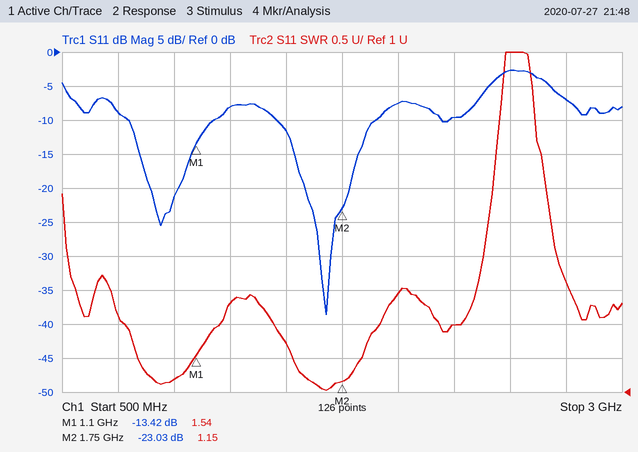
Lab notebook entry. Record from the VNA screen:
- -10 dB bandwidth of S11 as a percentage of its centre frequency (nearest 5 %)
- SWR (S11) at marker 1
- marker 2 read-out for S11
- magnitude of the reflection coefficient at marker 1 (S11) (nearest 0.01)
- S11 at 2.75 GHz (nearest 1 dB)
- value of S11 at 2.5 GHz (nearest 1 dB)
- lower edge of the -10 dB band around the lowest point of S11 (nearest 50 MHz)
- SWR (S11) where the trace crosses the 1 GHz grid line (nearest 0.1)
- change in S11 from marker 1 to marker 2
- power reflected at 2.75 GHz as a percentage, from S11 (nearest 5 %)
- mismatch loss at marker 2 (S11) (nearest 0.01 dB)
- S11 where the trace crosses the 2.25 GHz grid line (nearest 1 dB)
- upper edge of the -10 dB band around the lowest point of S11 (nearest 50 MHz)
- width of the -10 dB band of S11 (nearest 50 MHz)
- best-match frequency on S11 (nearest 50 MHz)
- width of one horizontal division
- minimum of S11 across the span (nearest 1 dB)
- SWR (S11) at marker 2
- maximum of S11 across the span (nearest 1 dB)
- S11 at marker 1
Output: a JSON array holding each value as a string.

["25 %", "1.54", "-23.03 dB", "0.21", "-7 dB", "-3 dB", "1.45 GHz", "1.2", "-9.61 dB", "20 %", "0.02 dB", "-10 dB", "1.90 GHz", "450 MHz", "1.70 GHz", "250 MHz", "-39 dB", "1.15", "-3 dB", "-13.42 dB"]
